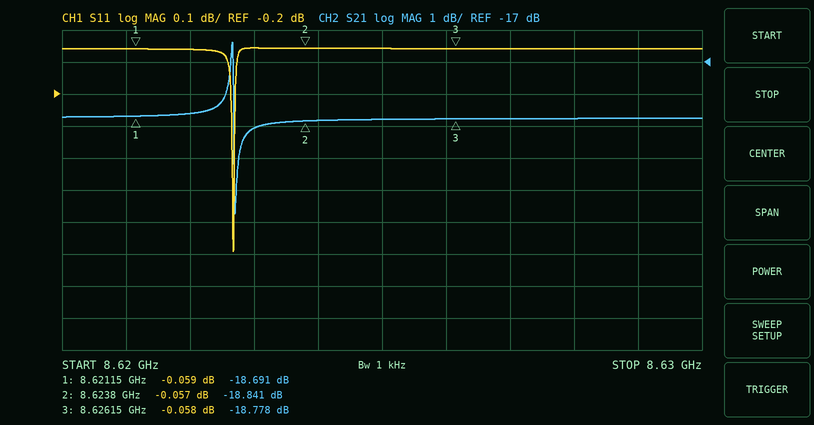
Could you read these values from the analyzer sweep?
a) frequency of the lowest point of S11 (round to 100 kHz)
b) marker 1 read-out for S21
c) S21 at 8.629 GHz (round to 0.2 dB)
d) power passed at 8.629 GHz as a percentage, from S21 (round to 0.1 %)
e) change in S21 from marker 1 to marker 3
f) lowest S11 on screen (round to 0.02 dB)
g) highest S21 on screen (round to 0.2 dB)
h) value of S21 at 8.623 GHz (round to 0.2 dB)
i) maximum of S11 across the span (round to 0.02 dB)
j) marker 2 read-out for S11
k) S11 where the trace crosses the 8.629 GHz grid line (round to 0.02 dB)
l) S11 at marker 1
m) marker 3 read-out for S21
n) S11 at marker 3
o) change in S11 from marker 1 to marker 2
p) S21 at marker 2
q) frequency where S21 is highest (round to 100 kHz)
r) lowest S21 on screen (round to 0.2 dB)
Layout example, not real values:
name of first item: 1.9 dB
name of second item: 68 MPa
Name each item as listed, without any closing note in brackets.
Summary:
frequency of the lowest point of S11: 8.6227 GHz
marker 1 read-out for S21: -18.691 dB
S21 at 8.629 GHz: -18.8 dB
power passed at 8.629 GHz as a percentage, from S21: 1.3 %
change in S21 from marker 1 to marker 3: -0.087 dB
lowest S11 on screen: -0.70 dB
highest S21 on screen: -16.4 dB
value of S21 at 8.623 GHz: -19.0 dB
maximum of S11 across the span: -0.06 dB
marker 2 read-out for S11: -0.057 dB
S11 where the trace crosses the 8.629 GHz grid line: -0.06 dB
S11 at marker 1: -0.059 dB
marker 3 read-out for S21: -18.778 dB
S11 at marker 3: -0.058 dB
change in S11 from marker 1 to marker 2: 0.002 dB
S21 at marker 2: -18.841 dB
frequency where S21 is highest: 8.6227 GHz
lowest S21 on screen: -21.8 dB
